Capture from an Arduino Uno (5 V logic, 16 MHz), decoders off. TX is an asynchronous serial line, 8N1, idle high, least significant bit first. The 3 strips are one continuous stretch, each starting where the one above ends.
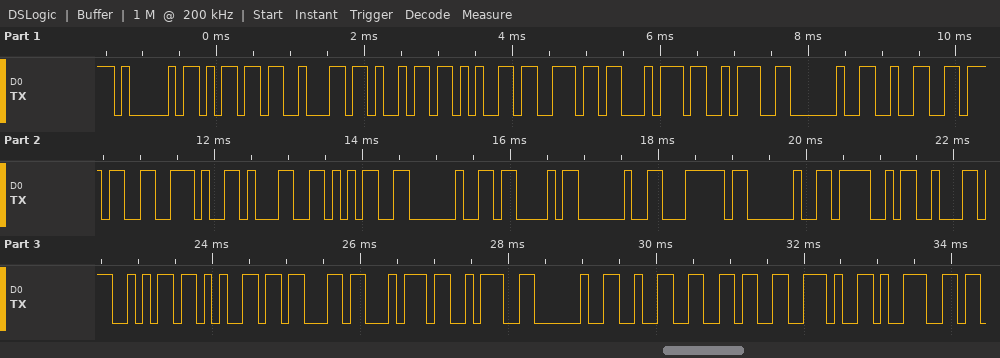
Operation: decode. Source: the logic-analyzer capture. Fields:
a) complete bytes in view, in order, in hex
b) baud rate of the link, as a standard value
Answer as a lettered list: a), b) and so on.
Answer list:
a) 41 6D 62 69 65 6E 74 3A 20 32 37 2E 31 35 20 43 20 7C 20 4F 62 6A 65 63 74 3A 20 32 36 2E 39
b) 9600 baud
